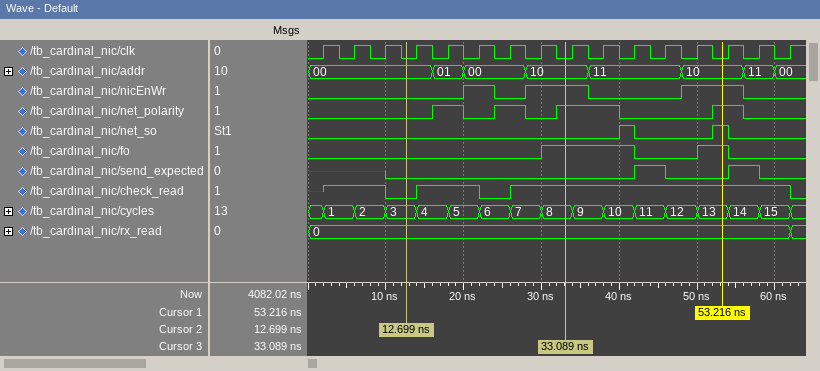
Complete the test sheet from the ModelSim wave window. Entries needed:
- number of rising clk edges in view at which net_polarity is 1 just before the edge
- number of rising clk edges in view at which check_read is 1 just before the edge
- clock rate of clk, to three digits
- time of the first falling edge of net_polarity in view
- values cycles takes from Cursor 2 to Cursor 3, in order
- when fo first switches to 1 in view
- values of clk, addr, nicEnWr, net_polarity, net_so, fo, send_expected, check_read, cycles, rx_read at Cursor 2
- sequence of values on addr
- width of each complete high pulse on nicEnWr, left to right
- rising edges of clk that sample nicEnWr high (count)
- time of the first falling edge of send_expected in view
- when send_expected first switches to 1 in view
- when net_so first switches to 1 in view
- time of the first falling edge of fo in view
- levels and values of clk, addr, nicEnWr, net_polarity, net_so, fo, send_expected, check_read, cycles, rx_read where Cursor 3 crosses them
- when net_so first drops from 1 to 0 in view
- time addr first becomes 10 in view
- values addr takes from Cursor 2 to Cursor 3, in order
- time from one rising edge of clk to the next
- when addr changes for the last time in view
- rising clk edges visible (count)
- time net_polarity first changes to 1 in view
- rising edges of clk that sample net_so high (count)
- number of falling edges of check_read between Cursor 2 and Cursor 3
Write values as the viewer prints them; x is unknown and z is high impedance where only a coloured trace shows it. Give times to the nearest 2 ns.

5
13
250 MHz
20 ns
3, 4, 5, 6, 7, 8
30 ns
clk=0, addr=00, nicEnWr=0, net_polarity=0, net_so=0, fo=0, send_expected=0, check_read=0, cycles=3, rx_read=0
00, 01, 00, 10, 11, 10, 11, 00
4 ns, 8 ns, 8 ns
5
46 ns
42 ns
40 ns
42 ns
clk=0, addr=10, nicEnWr=1, net_polarity=1, net_so=0, fo=1, send_expected=0, check_read=1, cycles=8, rx_read=0
42 ns
28 ns
00, 01, 00, 10
4 ns
60 ns
16
16 ns
2
1
